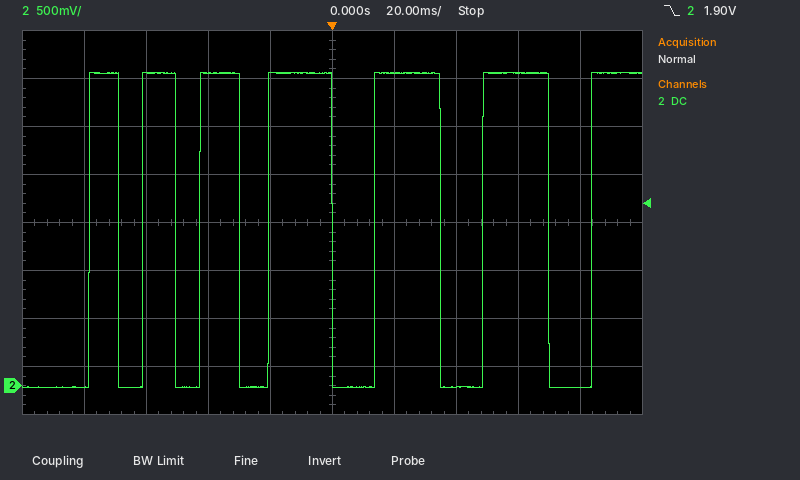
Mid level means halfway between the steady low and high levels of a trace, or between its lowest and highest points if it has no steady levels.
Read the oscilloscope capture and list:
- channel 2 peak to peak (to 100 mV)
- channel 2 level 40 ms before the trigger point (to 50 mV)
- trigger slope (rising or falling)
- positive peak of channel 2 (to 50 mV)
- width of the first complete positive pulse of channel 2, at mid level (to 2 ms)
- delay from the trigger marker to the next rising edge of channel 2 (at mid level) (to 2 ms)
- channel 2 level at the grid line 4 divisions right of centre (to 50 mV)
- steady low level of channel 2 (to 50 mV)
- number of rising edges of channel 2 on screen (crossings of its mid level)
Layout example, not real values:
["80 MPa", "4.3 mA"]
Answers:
["3.30 V", "3.25 V", "falling", "3.25 V", "10 ms", "14 ms", "0 mV", "0 mV", "7"]
